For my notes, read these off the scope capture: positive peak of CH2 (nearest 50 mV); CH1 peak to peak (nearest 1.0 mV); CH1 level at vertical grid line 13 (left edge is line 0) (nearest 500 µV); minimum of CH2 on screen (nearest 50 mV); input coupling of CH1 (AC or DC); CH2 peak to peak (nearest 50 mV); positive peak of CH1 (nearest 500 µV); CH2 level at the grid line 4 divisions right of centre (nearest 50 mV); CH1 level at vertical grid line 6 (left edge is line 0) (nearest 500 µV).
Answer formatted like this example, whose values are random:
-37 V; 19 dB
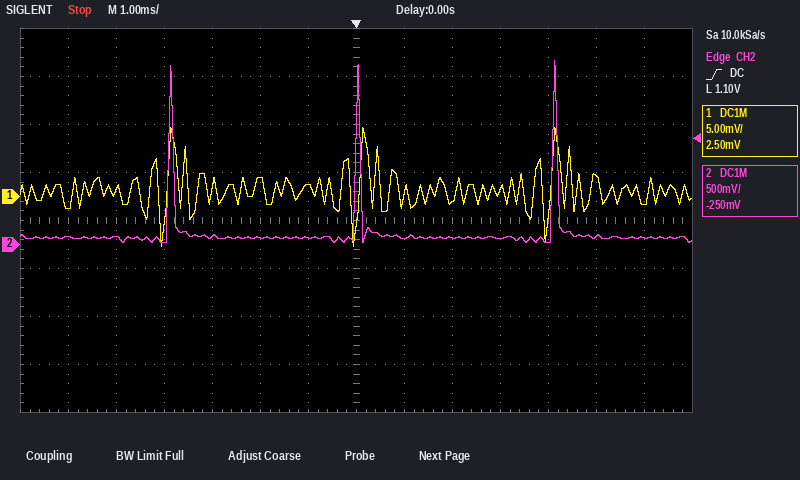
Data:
1.90 V; 12.0 mV; -1.0 mV; 0 mV; DC; 1.90 V; 7.0 mV; 0 mV; 1.0 mV
